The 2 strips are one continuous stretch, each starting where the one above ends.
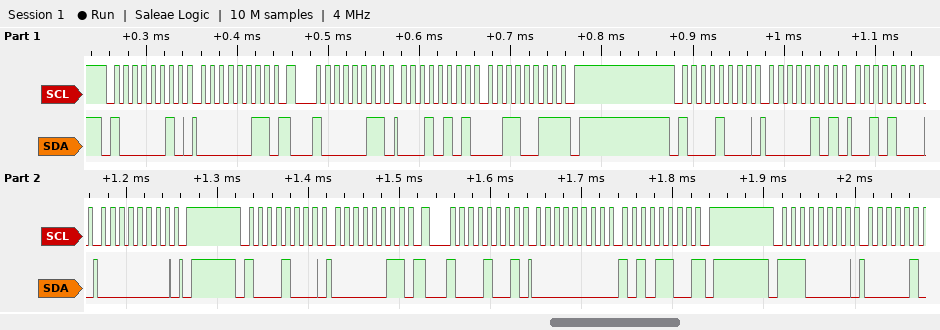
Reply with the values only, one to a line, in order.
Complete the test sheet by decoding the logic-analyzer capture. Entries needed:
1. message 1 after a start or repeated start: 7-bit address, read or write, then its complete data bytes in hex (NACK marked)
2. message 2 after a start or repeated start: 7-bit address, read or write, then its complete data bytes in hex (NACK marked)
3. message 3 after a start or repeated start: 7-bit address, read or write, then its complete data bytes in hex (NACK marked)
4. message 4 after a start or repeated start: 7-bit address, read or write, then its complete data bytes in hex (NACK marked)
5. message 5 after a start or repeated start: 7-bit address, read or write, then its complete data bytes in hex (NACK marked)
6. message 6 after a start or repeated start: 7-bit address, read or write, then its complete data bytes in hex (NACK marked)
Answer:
0x41 write: 03
0x41 read: 15 33 NACK
0x44 write: 05 28 00
0x44 write: 03
0x44 read: 00 AC NACK
0x70 write
